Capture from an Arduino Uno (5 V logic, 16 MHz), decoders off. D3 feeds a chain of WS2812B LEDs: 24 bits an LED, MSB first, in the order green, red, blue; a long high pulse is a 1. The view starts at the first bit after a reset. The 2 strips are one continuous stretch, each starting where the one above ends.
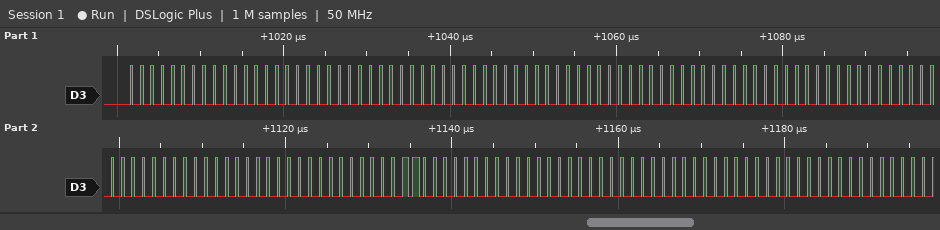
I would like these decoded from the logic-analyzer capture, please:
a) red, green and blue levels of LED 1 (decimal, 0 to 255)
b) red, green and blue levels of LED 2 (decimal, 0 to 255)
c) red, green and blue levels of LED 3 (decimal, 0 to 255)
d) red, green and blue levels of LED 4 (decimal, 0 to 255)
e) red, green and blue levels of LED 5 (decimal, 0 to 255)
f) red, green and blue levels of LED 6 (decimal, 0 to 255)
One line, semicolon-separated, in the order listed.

0, 0, 0; 0, 0, 0; 0, 0, 0; 0, 0, 0; 48, 0, 0; 0, 0, 0
